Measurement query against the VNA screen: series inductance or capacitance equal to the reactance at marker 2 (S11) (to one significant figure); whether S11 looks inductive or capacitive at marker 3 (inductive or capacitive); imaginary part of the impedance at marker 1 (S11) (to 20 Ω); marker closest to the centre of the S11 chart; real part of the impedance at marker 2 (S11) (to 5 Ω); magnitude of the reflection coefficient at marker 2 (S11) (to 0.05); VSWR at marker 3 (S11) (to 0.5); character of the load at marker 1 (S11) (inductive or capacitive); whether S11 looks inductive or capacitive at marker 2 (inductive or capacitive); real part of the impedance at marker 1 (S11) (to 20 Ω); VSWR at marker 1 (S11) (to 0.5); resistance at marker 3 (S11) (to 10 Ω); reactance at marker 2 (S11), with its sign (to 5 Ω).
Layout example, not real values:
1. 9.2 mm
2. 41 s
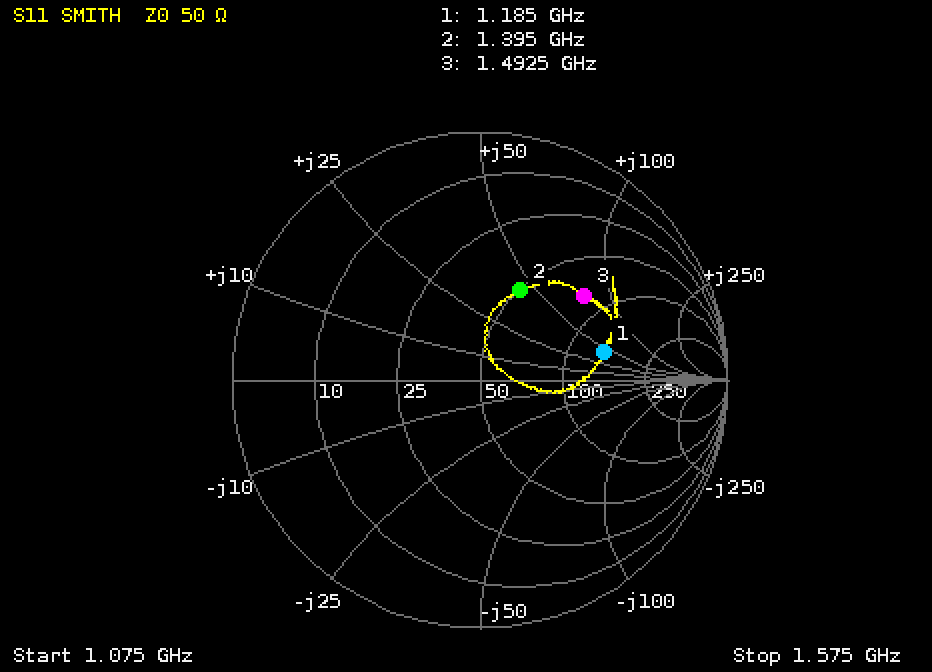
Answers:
1. 5 nH
2. inductive
3. +40 Ω
4. marker 2
5. 50 Ω
6. 0.40
7. 3.5
8. inductive
9. inductive
10. 140 Ω
11. 3.0
12. 80 Ω
13. +45 Ω
